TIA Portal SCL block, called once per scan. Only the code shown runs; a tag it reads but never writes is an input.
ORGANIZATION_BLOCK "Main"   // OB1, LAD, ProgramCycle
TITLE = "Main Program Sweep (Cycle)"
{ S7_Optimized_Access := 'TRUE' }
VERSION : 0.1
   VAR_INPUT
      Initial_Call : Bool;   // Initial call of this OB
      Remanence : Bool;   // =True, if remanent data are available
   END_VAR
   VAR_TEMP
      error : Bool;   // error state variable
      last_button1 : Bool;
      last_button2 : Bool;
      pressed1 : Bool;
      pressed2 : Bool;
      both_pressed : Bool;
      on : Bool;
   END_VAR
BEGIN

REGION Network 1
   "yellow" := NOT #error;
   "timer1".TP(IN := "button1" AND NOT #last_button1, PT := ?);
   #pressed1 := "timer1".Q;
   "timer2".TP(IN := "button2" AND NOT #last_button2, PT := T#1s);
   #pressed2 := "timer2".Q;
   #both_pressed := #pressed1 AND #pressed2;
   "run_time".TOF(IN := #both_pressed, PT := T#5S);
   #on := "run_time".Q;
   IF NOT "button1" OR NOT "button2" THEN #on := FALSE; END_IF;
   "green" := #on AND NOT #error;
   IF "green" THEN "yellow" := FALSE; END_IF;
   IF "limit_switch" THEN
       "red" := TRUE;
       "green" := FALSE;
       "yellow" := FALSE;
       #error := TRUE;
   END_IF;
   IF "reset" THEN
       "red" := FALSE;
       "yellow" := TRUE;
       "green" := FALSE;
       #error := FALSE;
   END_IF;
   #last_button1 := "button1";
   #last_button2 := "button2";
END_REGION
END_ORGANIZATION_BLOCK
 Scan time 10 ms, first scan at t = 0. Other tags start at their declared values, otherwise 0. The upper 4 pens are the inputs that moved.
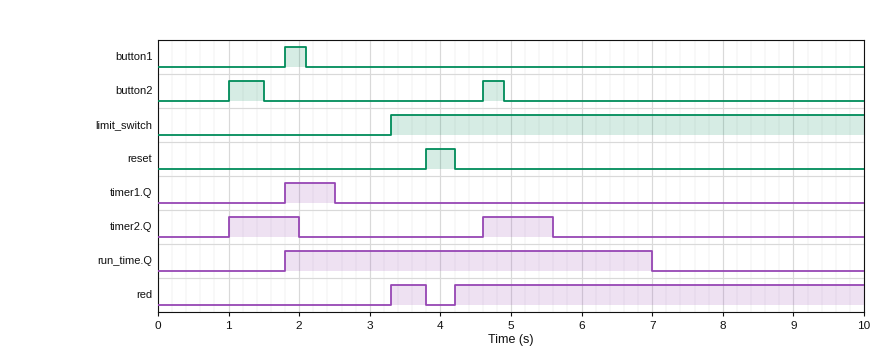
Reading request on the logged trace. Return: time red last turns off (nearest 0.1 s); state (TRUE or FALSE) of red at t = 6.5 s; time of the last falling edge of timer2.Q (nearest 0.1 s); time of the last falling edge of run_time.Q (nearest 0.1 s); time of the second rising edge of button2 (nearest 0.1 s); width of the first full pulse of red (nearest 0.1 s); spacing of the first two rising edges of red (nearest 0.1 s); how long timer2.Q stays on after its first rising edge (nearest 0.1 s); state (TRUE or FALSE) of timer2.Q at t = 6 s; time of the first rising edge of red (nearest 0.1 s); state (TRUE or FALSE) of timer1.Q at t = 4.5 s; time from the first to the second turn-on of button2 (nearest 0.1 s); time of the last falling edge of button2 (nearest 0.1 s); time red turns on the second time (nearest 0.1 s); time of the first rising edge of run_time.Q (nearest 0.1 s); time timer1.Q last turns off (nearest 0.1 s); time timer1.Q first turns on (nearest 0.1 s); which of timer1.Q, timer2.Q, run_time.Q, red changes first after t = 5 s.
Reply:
3.8 s
TRUE
5.6 s
7.0 s
4.6 s
0.5 s
0.9 s
1.0 s
FALSE
3.3 s
FALSE
3.6 s
4.9 s
4.2 s
1.8 s
2.5 s
1.8 s
timer2.Q
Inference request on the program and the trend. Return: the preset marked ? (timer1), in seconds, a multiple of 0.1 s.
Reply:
0.7 s
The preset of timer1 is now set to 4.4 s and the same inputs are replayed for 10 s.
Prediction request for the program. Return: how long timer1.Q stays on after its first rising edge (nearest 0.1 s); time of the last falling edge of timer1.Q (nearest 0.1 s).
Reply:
4.4 s
6.2 s
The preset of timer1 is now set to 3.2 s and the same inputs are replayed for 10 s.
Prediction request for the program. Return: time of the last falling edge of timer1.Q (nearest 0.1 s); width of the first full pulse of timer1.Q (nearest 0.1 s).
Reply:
5.0 s
3.2 s
